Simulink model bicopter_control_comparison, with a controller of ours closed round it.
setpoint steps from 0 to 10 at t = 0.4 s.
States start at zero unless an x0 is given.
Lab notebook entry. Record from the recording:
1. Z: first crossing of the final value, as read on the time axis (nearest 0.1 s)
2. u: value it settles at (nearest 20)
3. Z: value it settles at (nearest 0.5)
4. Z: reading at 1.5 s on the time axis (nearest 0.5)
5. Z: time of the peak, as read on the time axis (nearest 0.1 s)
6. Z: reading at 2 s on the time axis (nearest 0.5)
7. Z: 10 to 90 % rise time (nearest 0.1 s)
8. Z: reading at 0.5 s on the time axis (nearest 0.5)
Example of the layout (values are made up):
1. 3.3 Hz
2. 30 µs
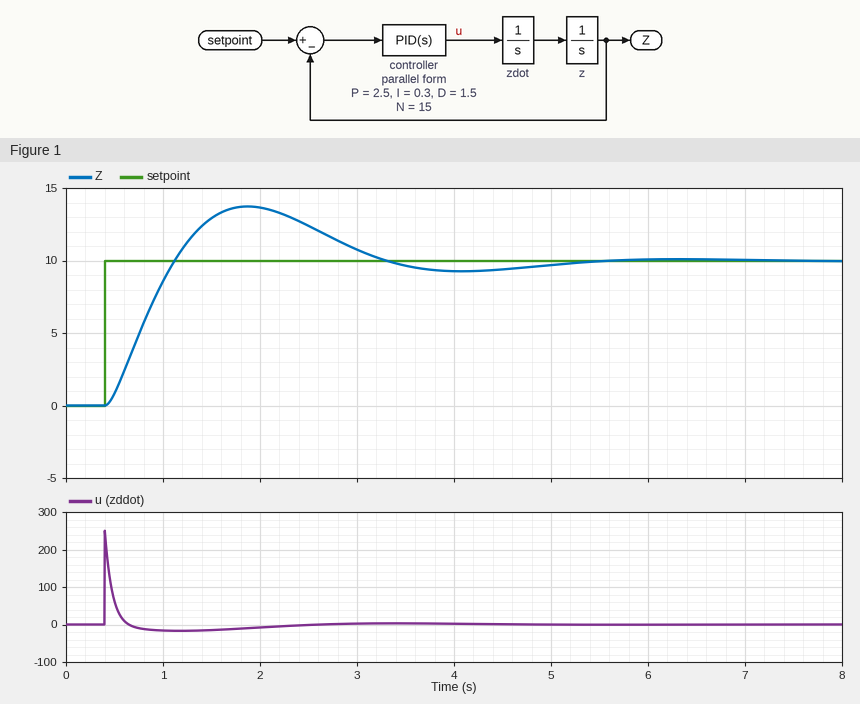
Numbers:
1. 1.1 s
2. 0
3. 10.0
4. 13.0
5. 1.9 s
6. 13.5
7. 0.5 s
8. 1.0
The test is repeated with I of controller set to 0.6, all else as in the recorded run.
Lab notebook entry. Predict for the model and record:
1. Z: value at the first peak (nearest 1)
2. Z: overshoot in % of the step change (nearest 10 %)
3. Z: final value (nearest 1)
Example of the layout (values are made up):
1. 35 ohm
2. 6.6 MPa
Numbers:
1. 14
2. 40 %
3. 10
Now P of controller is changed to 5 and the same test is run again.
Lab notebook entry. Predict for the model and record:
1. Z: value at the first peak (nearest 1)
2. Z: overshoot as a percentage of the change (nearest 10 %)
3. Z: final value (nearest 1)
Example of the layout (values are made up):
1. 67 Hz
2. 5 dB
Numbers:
1. 15
2. 50 %
3. 10
